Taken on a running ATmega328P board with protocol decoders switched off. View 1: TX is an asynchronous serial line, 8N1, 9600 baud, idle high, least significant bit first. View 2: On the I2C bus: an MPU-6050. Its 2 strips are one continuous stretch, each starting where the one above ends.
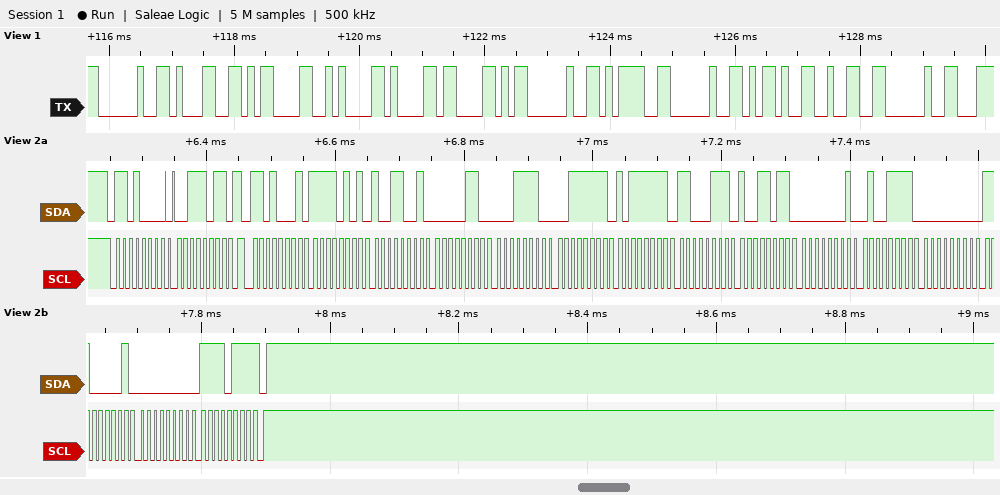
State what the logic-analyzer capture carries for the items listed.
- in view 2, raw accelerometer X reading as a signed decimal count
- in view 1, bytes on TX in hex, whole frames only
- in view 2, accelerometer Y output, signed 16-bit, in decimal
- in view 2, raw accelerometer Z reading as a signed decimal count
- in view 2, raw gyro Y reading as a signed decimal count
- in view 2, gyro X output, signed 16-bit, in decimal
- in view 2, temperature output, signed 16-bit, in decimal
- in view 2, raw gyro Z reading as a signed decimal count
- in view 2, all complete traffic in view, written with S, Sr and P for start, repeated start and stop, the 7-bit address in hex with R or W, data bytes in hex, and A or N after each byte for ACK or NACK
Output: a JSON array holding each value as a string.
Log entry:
["-2663", "20 31 0D 0A 61 58 20 3D 20 2D 32 20", "1566", "16319", "193", "335", "-14437", "247", "S 68W A 3B A Sr 68R A F5 A 99 A 06 A 1E A 3F A BF A C7 A 9B A 01 A 4F A 00 A C1 A 00 A F7 N P"]
